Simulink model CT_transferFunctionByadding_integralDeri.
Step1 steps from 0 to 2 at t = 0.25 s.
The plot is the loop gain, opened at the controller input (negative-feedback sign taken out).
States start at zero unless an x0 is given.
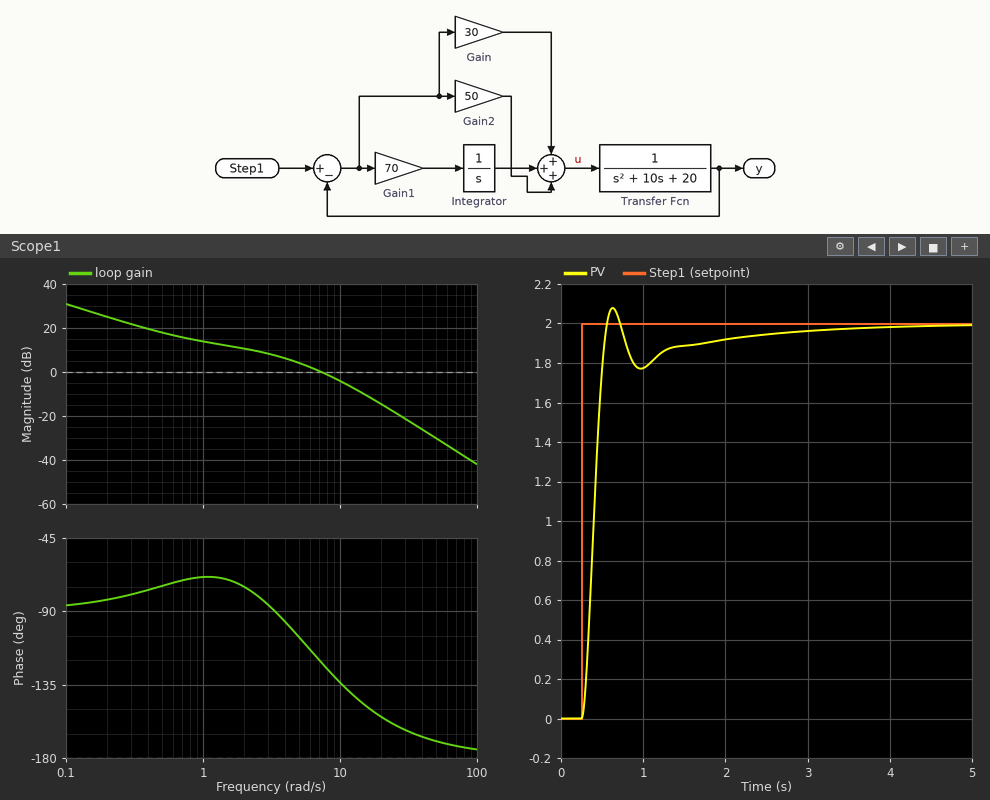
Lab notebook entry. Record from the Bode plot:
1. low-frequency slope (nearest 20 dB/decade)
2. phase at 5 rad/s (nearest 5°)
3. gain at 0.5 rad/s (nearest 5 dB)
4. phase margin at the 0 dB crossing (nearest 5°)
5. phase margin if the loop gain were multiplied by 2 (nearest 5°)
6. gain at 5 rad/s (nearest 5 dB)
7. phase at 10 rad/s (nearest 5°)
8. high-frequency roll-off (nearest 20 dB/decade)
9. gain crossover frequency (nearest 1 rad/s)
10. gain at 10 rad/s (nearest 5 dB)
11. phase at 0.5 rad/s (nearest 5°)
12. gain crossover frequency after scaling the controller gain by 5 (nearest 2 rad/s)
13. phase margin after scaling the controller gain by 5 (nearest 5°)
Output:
-20 dB/decade
-105°
20 dB
60°
40°
5 dB
-135°
-40 dB/decade
7 rad/s
-5 dB
-75°
20 rad/s
25°
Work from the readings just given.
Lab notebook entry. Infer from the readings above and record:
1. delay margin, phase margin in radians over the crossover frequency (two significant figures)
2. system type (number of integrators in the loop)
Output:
0.15 s
1
